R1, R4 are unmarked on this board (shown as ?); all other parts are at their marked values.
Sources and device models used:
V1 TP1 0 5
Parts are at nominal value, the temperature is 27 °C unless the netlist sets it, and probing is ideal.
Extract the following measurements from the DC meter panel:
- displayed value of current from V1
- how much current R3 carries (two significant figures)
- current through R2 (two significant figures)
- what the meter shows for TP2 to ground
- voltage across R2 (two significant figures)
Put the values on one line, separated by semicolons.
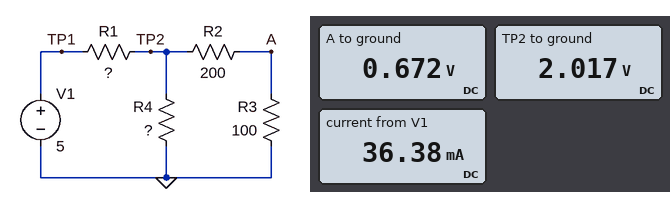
36.38 mA; 6.7 mA; 6.7 mA; 2.017 V; 1.3 V
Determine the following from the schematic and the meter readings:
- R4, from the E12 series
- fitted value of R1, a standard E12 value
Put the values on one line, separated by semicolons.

68 Ω; 82 Ω
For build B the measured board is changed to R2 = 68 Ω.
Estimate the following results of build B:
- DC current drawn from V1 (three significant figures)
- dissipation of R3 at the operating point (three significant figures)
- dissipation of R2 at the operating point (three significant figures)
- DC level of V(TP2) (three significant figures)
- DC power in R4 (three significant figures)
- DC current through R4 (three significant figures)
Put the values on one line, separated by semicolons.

38.3 mA; 12.2 mW; 8.30 mW; 1.86 V; 50.7 mW; 27.3 mA
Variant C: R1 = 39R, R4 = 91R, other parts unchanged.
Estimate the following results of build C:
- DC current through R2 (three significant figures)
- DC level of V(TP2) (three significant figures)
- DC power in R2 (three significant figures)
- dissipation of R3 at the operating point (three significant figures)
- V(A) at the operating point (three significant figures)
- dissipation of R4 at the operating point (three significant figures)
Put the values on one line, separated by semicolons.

10.7 mA; 3.21 V; 22.9 mW; 11.4 mW; 1.07 V; 113 mW
